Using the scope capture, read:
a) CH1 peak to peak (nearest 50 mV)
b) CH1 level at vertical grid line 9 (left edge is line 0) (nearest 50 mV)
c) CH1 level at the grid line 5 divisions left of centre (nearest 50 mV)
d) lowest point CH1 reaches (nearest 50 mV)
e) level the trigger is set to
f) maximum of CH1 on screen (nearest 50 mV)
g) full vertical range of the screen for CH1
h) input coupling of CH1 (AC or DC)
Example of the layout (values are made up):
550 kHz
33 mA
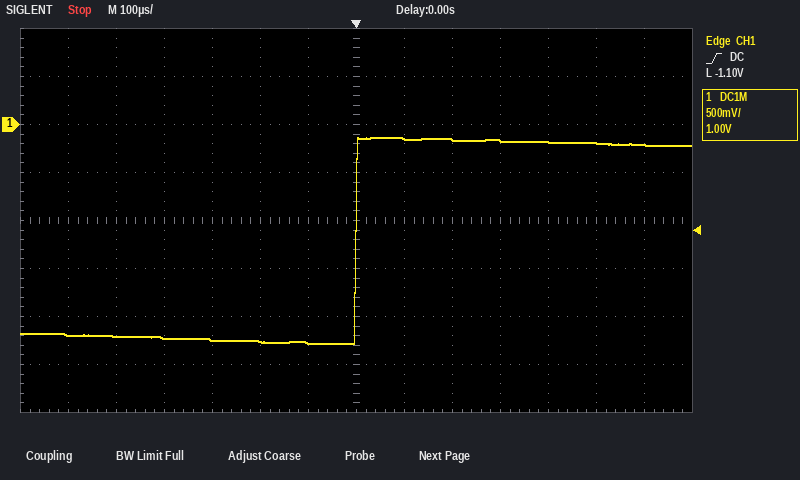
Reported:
2.15 V
-150 mV
-2.20 V
-2.30 V
-1.10 V
-150 mV
4 V
DC
